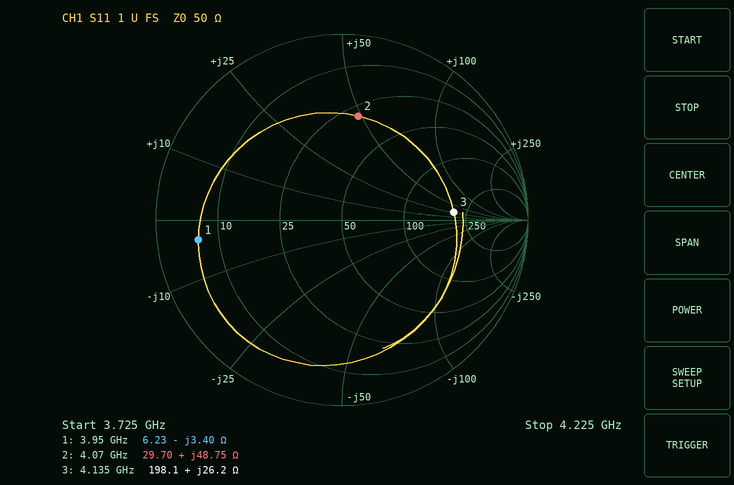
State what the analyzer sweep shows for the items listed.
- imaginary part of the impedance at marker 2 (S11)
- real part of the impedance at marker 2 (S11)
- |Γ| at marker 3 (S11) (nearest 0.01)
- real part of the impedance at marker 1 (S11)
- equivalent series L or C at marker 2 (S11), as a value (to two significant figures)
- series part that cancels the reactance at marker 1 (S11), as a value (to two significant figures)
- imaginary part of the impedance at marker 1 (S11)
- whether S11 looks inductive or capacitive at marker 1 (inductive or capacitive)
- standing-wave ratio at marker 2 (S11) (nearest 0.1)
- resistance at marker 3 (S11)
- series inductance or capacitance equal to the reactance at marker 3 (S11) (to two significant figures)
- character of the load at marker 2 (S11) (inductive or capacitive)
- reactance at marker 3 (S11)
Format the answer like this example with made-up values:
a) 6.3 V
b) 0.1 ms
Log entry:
a) +48.75 Ω
b) 29.70 Ω
c) 0.60
d) 6.23 Ω
e) 1.9 nH
f) 140 pH
g) -3.40 Ω
h) capacitive
i) 3.6
j) 198.1 Ω
k) 1.0 nH
l) inductive
m) +26.2 Ω
